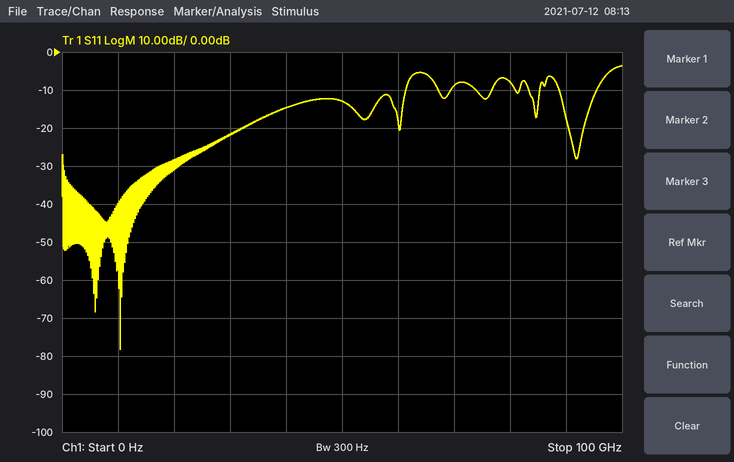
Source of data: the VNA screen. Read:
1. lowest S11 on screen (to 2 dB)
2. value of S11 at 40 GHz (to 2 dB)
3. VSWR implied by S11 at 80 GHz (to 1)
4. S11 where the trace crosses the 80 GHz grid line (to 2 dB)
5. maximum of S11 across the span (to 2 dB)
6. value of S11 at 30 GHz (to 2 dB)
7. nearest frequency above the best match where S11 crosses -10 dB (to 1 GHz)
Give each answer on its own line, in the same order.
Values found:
-78 dB
-14 dB
2
-8 dB
-4 dB
-22 dB
61 GHz
